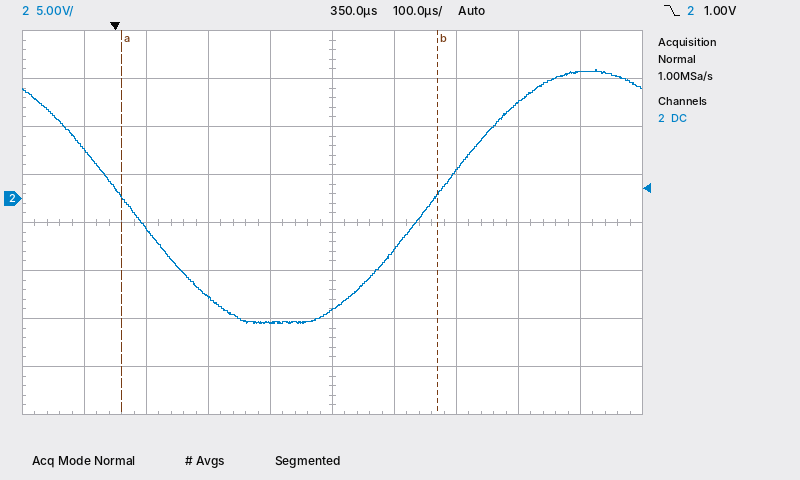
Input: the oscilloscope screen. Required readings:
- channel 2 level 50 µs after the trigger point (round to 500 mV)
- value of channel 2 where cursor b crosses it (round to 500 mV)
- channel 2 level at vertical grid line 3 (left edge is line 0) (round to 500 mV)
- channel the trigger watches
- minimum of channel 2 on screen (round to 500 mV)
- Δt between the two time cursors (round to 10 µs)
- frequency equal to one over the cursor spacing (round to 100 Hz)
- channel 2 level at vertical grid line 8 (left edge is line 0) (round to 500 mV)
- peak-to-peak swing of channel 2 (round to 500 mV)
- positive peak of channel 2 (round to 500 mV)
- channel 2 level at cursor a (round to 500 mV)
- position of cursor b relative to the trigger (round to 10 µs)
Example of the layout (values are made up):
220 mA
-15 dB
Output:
-3.0 V
500 mV
-10.5 V
channel 2
-13.0 V
510 µs
2.0 kHz
10.0 V
26.5 V
13.5 V
0.0 V
+520 µs
